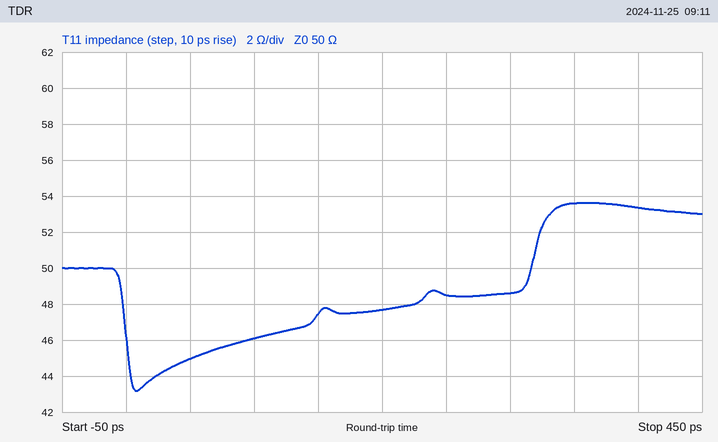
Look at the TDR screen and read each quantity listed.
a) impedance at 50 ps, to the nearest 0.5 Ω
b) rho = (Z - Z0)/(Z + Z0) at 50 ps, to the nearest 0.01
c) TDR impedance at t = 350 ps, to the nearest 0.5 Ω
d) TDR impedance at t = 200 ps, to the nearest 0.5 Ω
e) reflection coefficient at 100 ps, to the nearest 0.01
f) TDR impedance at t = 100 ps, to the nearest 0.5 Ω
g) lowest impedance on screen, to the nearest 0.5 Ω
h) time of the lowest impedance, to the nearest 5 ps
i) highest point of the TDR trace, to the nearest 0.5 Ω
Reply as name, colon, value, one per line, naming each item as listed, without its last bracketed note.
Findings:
impedance at 50 ps, to the nearest 0.5 Ω: 45.0 Ω
rho = (Z - Z0)/(Z + Z0) at 50 ps, to the nearest 0.01: -0.05
TDR impedance at t = 350 ps, to the nearest 0.5 Ω: 53.5 Ω
TDR impedance at t = 200 ps, to the nearest 0.5 Ω: 47.5 Ω
reflection coefficient at 100 ps, to the nearest 0.01: -0.04
TDR impedance at t = 100 ps, to the nearest 0.5 Ω: 46.0 Ω
lowest impedance on screen, to the nearest 0.5 Ω: 43.0 Ω
time of the lowest impedance, to the nearest 5 ps: 10 ps
highest point of the TDR trace, to the nearest 0.5 Ω: 53.5 Ω
